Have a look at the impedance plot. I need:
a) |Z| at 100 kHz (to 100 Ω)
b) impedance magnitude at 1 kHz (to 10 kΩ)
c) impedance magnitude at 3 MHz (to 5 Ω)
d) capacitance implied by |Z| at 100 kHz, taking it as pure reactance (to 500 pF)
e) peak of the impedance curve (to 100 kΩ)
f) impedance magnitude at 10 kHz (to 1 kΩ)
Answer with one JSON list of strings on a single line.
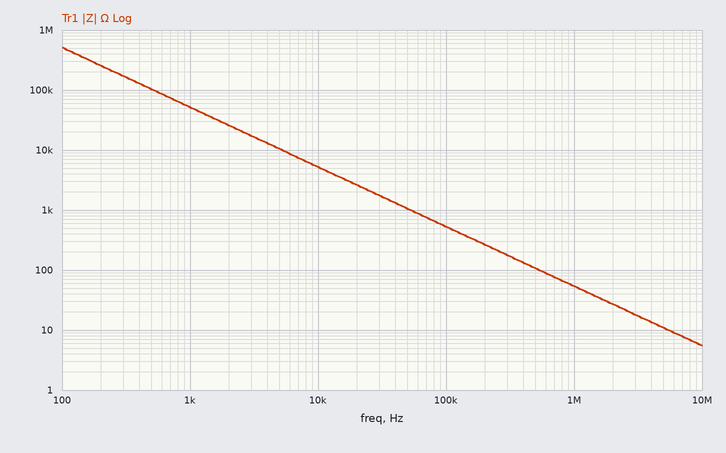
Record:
["500 Ω", "50 kΩ", "20 Ω", "3.0 nF", "500 kΩ", "5 kΩ"]
